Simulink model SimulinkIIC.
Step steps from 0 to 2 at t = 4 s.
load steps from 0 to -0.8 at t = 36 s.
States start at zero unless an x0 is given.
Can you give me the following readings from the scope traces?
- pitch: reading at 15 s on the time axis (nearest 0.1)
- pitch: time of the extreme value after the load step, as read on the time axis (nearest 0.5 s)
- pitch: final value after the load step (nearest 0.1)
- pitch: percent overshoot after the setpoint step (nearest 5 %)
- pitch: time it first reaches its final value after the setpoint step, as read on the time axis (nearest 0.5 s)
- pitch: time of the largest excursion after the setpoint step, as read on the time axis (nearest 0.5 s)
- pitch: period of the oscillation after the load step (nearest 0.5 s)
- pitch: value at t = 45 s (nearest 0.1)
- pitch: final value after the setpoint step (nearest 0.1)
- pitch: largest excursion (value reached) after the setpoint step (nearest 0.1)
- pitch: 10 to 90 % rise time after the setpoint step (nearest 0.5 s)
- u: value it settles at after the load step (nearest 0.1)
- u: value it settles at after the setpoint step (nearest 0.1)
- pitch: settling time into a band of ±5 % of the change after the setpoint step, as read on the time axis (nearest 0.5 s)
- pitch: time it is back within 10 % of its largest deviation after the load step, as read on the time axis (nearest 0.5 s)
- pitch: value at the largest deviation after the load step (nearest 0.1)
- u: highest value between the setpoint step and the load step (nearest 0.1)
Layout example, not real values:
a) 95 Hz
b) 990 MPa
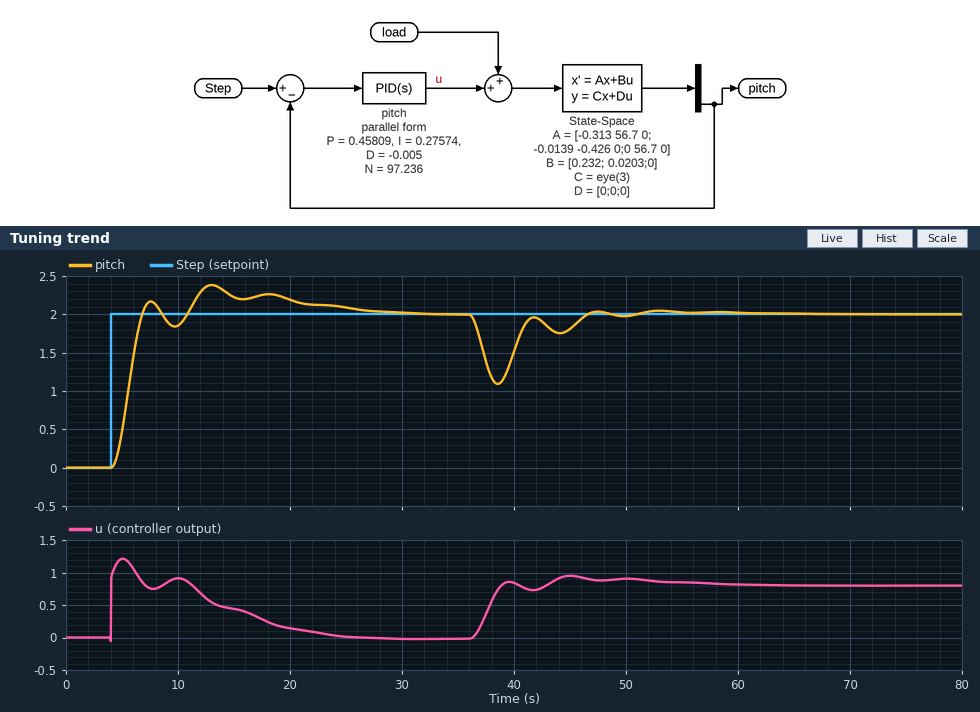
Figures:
a) 2.2
b) 38.5 s
c) 2.0
d) 20 %
e) 7.0 s
f) 13.0 s
g) 5.5 s
h) 1.8
i) 2.0
j) 2.4
k) 2.0 s
l) 0.8
m) 0.0
n) 24.5 s
o) 46.0 s
p) 1.1
q) 1.2
